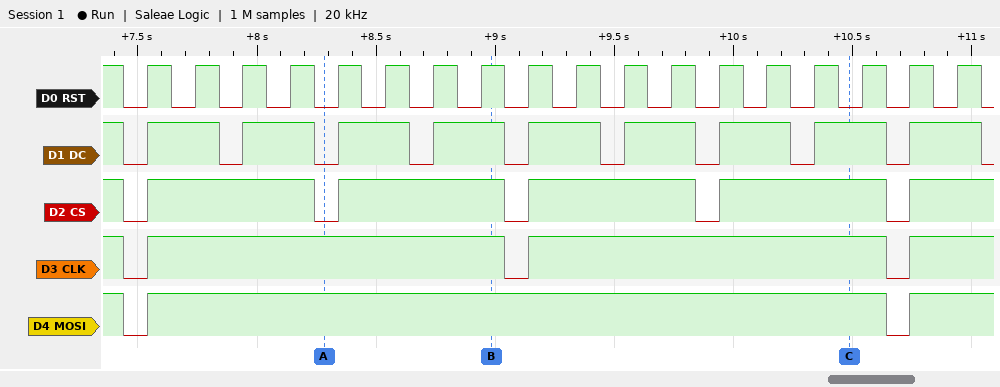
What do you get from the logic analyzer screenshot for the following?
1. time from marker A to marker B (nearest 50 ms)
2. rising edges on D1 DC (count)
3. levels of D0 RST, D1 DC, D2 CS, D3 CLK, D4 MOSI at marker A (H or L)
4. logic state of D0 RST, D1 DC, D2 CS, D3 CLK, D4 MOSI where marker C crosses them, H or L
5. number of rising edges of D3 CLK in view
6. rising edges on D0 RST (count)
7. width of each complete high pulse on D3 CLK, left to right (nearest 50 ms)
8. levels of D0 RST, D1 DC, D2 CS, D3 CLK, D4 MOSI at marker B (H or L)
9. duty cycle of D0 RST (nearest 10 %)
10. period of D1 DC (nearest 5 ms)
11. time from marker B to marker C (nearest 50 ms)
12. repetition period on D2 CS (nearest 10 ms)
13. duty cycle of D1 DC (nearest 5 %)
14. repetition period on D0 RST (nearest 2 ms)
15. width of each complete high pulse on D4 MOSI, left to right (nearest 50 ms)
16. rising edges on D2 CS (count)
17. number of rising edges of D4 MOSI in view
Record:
700 ms
9
D0 RST=L, D1 DC=L, D2 CS=L, D3 CLK=H, D4 MOSI=H
D0 RST=L, D1 DC=H, D2 CS=H, D3 CLK=H, D4 MOSI=H
3
18
1500 ms, 1500 ms
D0 RST=H, D1 DC=H, D2 CS=H, D3 CLK=H, D4 MOSI=H
50 %
400 ms
1500 ms
800 ms
75 %
200 ms
3100 ms
5
2
